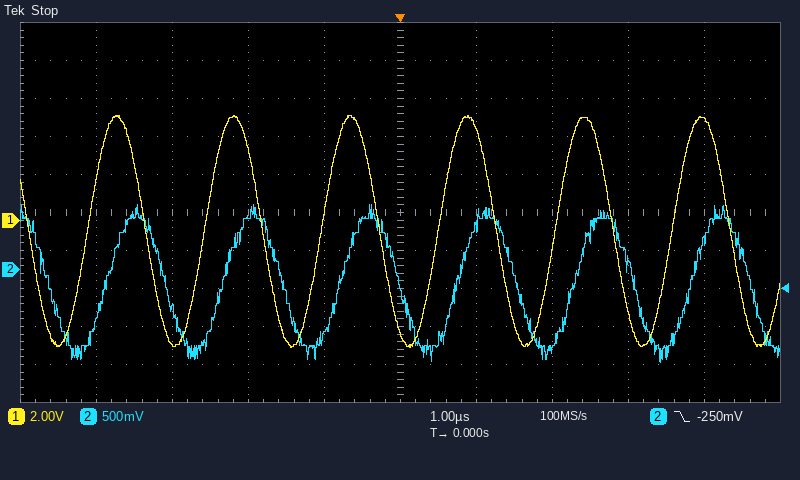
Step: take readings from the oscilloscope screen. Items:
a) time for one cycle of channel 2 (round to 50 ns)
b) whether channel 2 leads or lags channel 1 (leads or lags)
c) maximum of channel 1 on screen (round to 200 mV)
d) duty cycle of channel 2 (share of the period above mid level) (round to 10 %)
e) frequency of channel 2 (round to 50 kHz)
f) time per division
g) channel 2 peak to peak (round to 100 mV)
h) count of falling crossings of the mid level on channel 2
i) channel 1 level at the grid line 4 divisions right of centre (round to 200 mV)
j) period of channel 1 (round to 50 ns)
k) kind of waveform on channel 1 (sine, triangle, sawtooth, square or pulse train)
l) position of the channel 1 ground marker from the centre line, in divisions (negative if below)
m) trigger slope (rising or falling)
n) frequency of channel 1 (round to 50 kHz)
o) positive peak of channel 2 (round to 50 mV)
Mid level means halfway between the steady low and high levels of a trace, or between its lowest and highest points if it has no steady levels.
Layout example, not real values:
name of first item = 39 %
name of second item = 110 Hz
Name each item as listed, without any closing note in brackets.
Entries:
time for one cycle of channel 2 = 1.55 µs
whether channel 2 leads or lags channel 1 = lags
maximum of channel 1 on screen = 5.6 V
duty cycle of channel 2 (share of the period above mid level) = 50 %
frequency of channel 2 = 650 kHz
time per division = 1 µs
channel 2 peak to peak = 2.10 V
count of falling crossings of the mid level on channel 2 = 7
channel 1 level at the grid line 4 divisions right of centre = 5.2 V
period of channel 1 = 1.55 µs
kind of waveform on channel 1 = sine
position of the channel 1 ground marker from the centre line, in divisions = -0.2 div
trigger slope = falling
frequency of channel 1 = 650 kHz
positive peak of channel 2 = 850 mV
